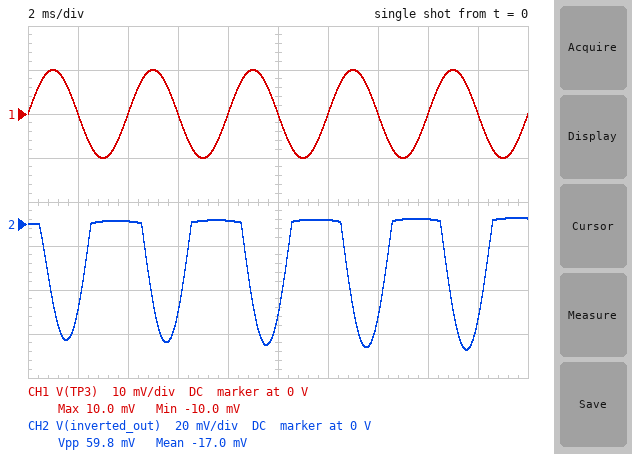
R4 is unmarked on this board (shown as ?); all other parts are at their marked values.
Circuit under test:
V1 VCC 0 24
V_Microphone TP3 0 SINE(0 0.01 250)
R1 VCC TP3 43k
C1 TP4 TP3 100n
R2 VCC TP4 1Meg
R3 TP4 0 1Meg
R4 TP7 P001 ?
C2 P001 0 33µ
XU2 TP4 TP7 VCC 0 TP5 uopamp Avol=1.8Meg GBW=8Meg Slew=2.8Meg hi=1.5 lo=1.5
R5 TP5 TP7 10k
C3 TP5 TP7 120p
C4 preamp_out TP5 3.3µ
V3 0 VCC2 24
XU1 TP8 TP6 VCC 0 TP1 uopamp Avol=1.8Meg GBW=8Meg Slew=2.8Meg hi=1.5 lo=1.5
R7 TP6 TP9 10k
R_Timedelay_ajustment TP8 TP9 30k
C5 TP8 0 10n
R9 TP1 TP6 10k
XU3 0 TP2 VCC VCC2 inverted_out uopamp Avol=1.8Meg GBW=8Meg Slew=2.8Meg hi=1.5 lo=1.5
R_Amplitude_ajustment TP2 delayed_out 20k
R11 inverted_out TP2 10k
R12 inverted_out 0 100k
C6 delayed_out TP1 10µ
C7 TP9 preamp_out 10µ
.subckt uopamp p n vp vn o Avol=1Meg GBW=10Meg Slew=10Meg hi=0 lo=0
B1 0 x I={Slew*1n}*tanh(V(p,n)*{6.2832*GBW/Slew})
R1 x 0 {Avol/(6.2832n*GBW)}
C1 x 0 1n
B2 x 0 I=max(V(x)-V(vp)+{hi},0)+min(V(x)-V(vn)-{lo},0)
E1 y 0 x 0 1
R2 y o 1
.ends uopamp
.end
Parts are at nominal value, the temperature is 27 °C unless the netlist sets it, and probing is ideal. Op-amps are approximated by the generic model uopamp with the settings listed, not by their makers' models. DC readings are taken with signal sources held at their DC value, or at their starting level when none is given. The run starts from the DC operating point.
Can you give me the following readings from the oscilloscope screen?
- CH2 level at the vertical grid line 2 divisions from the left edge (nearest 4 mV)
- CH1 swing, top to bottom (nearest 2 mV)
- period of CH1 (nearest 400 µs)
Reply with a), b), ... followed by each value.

a) 0 V
b) 20 mV
c) 4.0 ms
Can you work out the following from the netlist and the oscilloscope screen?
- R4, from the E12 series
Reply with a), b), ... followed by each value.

a) 1 kΩ
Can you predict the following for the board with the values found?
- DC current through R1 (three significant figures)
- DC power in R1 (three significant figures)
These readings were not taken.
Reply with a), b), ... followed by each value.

a) 558 µA
b) 13.4 mW
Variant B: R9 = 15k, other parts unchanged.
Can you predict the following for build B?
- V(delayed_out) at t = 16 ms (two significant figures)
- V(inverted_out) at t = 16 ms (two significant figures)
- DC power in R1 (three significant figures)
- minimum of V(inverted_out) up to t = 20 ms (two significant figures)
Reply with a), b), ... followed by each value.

a) -4.6 mV
b) 2.3 mV
c) 13.4 mW
d) -62 mV
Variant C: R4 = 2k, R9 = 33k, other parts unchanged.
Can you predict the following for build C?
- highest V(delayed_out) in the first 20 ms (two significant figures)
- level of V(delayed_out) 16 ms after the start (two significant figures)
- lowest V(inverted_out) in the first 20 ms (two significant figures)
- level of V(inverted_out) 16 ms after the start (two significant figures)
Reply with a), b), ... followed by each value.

a) 100 mV
b) -3.5 mV
c) -50 mV
d) 1.7 mV
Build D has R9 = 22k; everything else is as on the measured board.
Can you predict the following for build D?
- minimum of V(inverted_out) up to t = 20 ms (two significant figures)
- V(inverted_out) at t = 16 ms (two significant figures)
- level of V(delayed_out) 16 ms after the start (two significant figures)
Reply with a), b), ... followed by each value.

a) -72 mV
b) 2.6 mV
c) -5.2 mV
